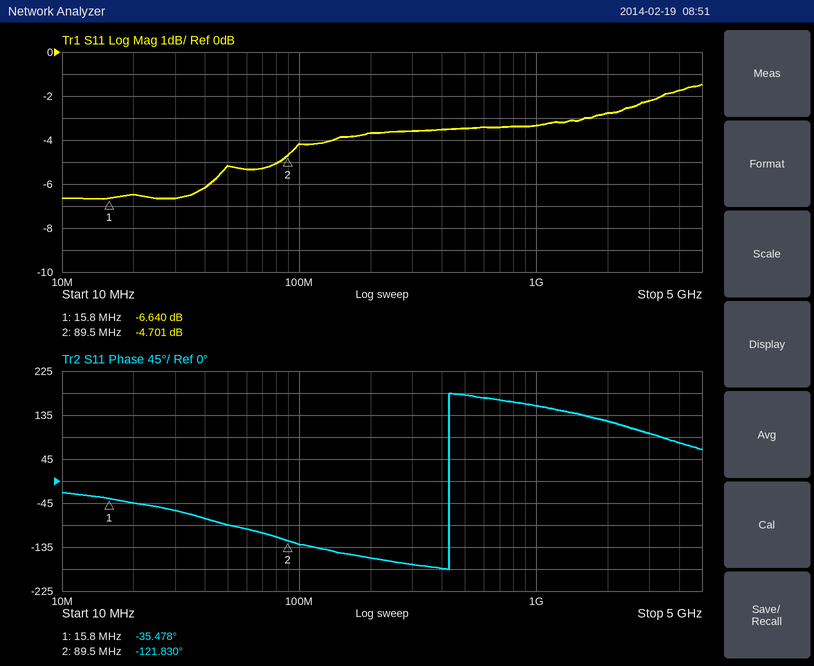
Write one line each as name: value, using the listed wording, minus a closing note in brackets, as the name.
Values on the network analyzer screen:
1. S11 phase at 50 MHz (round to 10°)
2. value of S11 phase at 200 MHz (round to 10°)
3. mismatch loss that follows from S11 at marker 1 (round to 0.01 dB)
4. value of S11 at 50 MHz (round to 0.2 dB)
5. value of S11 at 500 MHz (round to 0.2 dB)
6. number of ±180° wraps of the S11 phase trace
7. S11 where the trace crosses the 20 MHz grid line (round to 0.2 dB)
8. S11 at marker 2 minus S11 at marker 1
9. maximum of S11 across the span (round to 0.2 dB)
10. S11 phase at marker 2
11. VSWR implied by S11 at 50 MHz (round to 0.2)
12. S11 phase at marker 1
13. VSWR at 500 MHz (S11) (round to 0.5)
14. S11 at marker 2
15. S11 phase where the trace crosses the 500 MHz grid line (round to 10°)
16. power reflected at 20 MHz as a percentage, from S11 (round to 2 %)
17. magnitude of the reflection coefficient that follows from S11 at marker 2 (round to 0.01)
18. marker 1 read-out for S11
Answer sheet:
S11 phase at 50 MHz: -90°
value of S11 phase at 200 MHz: -160°
mismatch loss that follows from S11 at marker 1: 1.06 dB
value of S11 at 50 MHz: -5.2 dB
value of S11 at 500 MHz: -3.4 dB
number of ±180° wraps of the S11 phase trace: 1
S11 where the trace crosses the 20 MHz grid line: -6.4 dB
S11 at marker 2 minus S11 at marker 1: 1.939 dB
maximum of S11 across the span: -1.4 dB
S11 phase at marker 2: -121.830°
VSWR implied by S11 at 50 MHz: 3.4
S11 phase at marker 1: -35.478°
VSWR at 500 MHz (S11): 5.0
S11 at marker 2: -4.701 dB
S11 phase where the trace crosses the 500 MHz grid line: 180°
power reflected at 20 MHz as a percentage, from S11: 22 %
magnitude of the reflection coefficient that follows from S11 at marker 2: 0.58
marker 1 read-out for S11: -6.640 dB
